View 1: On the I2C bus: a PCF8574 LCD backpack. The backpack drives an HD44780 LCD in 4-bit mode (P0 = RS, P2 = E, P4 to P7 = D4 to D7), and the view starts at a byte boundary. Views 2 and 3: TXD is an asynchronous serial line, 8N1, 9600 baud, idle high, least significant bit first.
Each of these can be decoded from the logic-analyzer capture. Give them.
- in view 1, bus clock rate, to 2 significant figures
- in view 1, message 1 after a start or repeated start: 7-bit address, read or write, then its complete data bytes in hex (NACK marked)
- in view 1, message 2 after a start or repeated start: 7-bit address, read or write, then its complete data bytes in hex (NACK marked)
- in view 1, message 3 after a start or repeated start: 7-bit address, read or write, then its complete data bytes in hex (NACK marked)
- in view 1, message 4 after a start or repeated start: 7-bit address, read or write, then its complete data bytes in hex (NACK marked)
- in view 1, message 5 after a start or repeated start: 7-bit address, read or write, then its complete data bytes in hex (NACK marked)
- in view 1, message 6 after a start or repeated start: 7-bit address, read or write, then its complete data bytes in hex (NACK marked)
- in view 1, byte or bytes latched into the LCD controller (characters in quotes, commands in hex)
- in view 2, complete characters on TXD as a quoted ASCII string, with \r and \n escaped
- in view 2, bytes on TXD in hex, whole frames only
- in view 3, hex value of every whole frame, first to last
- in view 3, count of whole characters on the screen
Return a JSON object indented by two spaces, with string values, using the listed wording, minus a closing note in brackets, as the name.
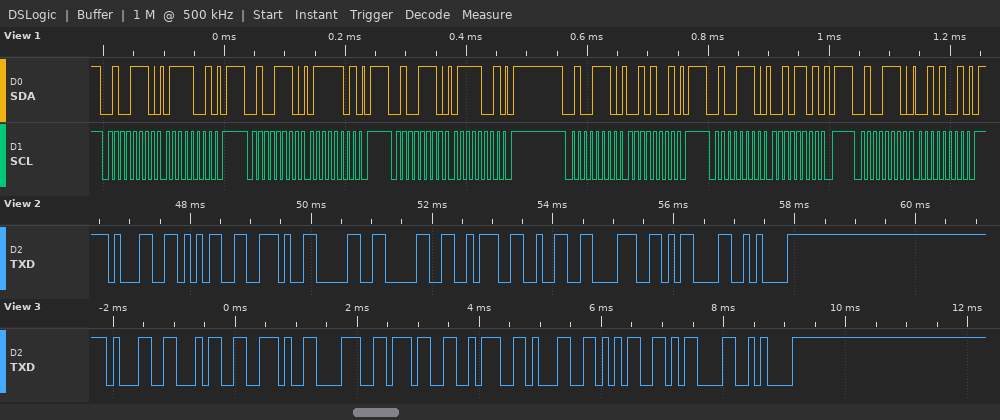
{
  "in view 1, bus clock rate, to 2 significant figures": "100 kHz",
  "in view 1, message 1 after a start or repeated start: 7-bit address, read or write, then its complete data bytes in hex": "0x27 write: 79",
  "in view 1, message 2 after a start or repeated start: 7-bit address, read or write, then its complete data bytes in hex": "0x27 write: 7D",
  "in view 1, message 3 after a start or repeated start: 7-bit address, read or write, then its complete data bytes in hex": "0x27 write: 79",
  "in view 1, message 4 after a start or repeated start: 7-bit address, read or write, then its complete data bytes in hex": "0x27 write: 29",
  "in view 1, message 5 after a start or repeated start: 7-bit address, read or write, then its complete data bytes in hex": "0x27 write: 2D",
  "in view 1, message 6 after a start or repeated start: 7-bit address, read or write, then its complete data bytes in hex": "0x27 write: 29",
  "in view 1, byte or bytes latched into the LCD controller": "'r'",
  "in view 2, complete characters on TXD as a quoted ASCII string, with \\r and \\n escaped": "\"15.00:28\\r\\n\"",
  "in view 2, bytes on TXD in hex, whole frames only": "31 35 2E 30 30 3A 32 38 0D 0A",
  "in view 3, hex value of every whole frame, first to last": "31 34 2E 38 37 3A 31 35 0D 0A",
  "in view 3, count of whole characters on the screen": "10"
}
